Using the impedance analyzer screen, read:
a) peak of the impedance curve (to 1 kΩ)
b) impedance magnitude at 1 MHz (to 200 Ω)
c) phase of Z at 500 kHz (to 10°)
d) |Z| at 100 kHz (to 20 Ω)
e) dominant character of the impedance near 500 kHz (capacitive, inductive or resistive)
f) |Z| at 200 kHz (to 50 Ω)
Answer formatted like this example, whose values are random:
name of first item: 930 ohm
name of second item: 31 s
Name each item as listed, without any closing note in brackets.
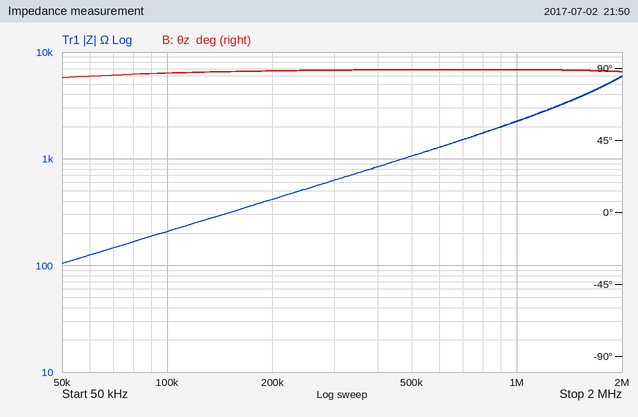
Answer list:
peak of the impedance curve: 6 kΩ
impedance magnitude at 1 MHz: 2.2 kΩ
phase of Z at 500 kHz: 90°
|Z| at 100 kHz: 200 Ω
dominant character of the impedance near 500 kHz: inductive
|Z| at 200 kHz: 400 Ω
